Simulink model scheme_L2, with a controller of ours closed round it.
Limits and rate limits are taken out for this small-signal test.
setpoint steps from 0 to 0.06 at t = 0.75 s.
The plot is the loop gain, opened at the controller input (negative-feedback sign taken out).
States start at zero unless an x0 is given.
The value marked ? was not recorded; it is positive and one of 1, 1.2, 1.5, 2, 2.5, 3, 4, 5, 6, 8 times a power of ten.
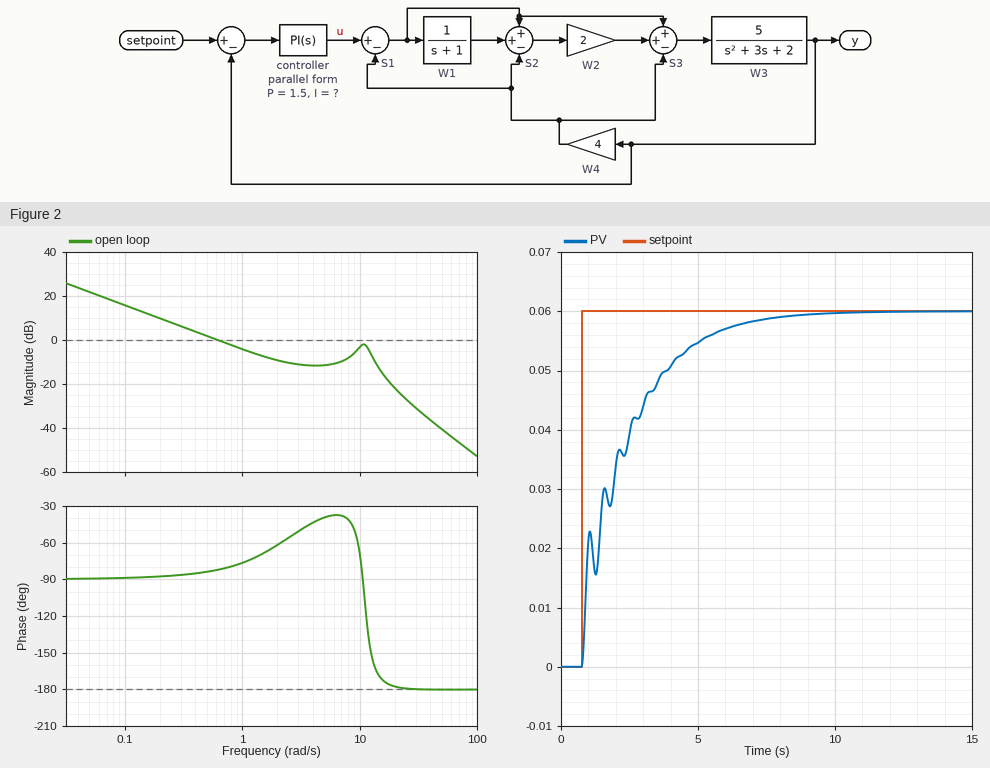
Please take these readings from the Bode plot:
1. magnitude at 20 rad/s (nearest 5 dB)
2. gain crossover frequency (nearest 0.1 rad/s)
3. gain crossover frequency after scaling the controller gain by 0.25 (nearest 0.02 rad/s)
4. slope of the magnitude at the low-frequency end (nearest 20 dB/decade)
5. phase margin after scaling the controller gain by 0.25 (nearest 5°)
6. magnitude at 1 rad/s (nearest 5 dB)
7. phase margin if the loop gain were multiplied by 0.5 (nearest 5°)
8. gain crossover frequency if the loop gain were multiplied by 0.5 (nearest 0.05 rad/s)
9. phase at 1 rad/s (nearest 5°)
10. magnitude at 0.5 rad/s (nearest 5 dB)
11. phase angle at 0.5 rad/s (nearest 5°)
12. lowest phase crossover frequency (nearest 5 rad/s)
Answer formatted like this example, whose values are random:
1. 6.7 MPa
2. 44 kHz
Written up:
1. -20 dB
2. 0.6 rad/s
3. 0.16 rad/s
4. -20 dB/decade
5. 90°
6. -5 dB
7. 95°
8. 0.30 rad/s
9. -75°
10. 0 dB
11. -85°
12. 35 rad/s
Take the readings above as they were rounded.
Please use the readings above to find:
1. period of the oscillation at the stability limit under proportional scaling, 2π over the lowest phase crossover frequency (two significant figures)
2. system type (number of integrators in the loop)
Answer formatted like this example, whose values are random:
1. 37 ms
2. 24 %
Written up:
1. 0.18 s
2. 1
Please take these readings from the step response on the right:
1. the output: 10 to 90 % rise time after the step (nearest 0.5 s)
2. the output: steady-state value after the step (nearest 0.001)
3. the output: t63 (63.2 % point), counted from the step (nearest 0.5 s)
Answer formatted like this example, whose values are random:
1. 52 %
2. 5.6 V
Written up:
1. 4.0 s
2. 0.060
3. 1.5 s
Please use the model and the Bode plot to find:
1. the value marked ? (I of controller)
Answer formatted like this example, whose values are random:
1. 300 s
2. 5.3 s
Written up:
1. 4
